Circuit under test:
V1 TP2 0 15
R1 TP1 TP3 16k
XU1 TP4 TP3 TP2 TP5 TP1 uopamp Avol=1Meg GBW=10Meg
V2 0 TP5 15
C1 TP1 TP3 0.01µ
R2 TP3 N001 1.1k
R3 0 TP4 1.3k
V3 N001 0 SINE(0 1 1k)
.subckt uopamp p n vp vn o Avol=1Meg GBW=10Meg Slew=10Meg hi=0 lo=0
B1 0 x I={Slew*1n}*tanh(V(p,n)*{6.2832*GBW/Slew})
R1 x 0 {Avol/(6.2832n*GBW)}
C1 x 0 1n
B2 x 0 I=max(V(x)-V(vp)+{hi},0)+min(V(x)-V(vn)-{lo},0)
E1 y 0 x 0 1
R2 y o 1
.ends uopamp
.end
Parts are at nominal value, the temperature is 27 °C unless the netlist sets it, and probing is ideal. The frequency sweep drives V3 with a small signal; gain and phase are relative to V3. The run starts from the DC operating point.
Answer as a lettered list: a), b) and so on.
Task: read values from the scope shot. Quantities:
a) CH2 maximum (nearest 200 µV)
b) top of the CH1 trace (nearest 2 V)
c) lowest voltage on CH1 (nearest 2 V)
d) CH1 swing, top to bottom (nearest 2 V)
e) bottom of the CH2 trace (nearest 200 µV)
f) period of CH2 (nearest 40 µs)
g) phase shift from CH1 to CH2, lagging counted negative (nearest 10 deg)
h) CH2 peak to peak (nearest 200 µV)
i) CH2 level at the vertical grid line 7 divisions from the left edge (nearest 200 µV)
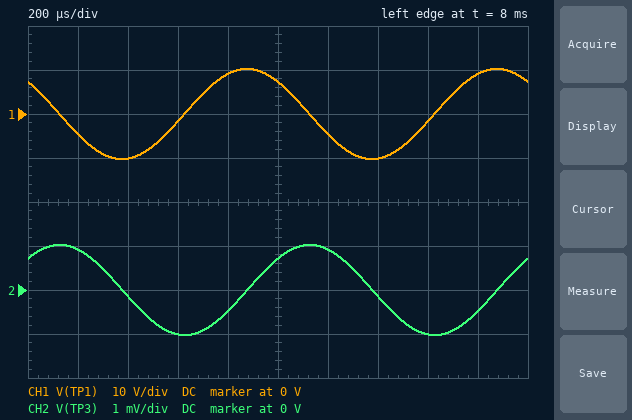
a) 1.0 mV
b) 10 V
c) -10 V
d) 20 V
e) -1.0 mV
f) 1.00 ms
g) -90 deg
h) 2.0 mV
i) -200 µV
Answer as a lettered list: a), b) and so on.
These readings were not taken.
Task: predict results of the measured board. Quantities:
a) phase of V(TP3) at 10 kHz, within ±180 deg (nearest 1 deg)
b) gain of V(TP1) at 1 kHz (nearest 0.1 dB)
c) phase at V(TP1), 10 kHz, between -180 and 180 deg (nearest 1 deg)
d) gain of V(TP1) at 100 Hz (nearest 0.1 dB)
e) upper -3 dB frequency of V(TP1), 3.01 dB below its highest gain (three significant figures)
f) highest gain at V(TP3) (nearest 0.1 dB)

a) 6 deg
b) 20.2 dB
c) 96 deg
d) 23.2 dB
e) 993 Hz
f) -56.8 dB
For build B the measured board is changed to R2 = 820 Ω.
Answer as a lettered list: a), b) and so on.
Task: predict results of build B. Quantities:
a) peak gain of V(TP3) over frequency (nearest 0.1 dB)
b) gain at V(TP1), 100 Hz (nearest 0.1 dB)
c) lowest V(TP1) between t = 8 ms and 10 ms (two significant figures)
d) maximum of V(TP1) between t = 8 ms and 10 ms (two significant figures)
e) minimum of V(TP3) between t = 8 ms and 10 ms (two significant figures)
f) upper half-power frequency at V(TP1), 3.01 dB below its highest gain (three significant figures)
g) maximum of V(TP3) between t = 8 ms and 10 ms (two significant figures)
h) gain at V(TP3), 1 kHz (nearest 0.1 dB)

a) -54.3 dB
b) 25.8 dB
c) -14 V
d) 14 V
e) -1.4 mV
f) 993 Hz
g) 1.4 mV
h) -57.2 dB
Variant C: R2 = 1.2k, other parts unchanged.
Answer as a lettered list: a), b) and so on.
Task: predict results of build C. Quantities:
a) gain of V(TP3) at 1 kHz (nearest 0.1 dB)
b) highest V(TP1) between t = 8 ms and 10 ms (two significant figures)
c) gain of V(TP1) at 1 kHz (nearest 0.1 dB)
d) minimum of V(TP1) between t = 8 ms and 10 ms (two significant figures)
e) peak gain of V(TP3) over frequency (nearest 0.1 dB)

a) -60.5 dB
b) 9.4 V
c) 19.5 dB
d) -9.4 V
e) -57.6 dB
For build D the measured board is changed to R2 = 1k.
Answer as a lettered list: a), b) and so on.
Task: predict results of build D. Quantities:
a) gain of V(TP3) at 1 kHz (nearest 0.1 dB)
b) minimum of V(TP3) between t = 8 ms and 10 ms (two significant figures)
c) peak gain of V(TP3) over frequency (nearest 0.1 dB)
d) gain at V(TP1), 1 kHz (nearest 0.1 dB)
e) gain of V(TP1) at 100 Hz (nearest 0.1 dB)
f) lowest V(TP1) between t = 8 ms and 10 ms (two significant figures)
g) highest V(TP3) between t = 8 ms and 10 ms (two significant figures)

a) -59.0 dB
b) -1.1 mV
c) -56.0 dB
d) 21.0 dB
e) 24.0 dB
f) -11 V
g) 1.1 mV
